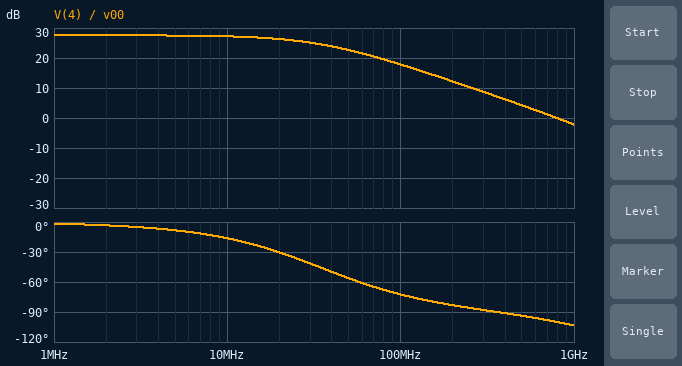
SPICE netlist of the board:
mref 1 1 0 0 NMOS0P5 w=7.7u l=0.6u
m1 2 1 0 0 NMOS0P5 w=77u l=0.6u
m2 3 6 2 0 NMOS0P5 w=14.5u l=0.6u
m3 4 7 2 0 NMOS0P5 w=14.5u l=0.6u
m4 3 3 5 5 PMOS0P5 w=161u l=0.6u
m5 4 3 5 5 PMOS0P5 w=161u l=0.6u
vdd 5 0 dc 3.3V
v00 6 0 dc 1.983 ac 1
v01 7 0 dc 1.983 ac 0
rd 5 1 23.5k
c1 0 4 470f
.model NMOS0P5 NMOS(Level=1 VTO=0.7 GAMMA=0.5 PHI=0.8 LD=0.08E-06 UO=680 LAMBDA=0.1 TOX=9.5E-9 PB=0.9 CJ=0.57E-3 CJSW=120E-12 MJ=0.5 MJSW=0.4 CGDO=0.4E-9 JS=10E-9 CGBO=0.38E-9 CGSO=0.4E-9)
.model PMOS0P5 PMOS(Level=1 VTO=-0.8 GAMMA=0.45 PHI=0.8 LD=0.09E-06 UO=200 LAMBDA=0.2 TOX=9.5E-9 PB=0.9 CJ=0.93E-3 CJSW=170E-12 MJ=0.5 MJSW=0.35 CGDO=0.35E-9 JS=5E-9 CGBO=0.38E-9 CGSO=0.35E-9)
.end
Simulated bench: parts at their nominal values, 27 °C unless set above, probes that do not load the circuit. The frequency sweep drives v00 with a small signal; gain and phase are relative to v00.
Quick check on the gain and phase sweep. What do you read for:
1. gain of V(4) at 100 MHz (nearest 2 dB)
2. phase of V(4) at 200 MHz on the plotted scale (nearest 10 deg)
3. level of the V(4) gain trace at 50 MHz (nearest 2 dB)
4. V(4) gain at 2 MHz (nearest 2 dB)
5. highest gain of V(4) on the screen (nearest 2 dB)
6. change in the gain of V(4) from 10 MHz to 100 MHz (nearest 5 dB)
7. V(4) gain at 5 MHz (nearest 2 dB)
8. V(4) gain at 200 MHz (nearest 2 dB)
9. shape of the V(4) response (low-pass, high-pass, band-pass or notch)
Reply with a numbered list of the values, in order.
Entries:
1. 18 dB
2. -80 deg
3. 22 dB
4. 28 dB
5. 28 dB
6. -10 dB
7. 28 dB
8. 12 dB
9. low-pass
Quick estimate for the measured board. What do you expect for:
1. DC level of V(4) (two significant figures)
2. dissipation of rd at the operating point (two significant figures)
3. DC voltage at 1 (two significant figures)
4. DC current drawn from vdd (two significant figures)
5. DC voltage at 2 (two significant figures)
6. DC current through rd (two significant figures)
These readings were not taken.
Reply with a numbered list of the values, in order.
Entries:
1. 2.3 V
2. 240 µW
3. 910 mV
4. 1.1 mA
5. 780 mV
6. 100 µA
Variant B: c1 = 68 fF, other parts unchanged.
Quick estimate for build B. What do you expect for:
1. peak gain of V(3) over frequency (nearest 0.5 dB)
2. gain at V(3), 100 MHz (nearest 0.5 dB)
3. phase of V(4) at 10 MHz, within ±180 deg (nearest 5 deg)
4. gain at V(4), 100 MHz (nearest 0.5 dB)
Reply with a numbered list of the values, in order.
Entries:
1. -15.0 dB
2. -16.5 dB
3. -5 deg
4. 25.0 dB
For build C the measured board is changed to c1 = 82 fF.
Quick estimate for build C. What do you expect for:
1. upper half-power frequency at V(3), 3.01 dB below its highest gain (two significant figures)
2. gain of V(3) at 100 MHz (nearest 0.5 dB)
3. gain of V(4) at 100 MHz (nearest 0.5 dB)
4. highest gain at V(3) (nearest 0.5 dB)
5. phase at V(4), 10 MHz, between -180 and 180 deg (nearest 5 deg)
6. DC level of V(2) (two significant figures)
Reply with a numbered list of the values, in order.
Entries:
1. 2.4 GHz
2. -16.5 dB
3. 24.5 dB
4. -15.0 dB
5. -5 deg
6. 780 mV
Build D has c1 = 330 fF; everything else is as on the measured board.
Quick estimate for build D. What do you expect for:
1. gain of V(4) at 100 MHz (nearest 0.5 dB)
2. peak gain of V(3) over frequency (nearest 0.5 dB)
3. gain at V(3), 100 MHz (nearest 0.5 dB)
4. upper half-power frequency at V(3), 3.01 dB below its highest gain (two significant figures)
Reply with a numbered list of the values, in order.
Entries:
1. 20.0 dB
2. -13.5 dB
3. -14.0 dB
4. 2.9 GHz
